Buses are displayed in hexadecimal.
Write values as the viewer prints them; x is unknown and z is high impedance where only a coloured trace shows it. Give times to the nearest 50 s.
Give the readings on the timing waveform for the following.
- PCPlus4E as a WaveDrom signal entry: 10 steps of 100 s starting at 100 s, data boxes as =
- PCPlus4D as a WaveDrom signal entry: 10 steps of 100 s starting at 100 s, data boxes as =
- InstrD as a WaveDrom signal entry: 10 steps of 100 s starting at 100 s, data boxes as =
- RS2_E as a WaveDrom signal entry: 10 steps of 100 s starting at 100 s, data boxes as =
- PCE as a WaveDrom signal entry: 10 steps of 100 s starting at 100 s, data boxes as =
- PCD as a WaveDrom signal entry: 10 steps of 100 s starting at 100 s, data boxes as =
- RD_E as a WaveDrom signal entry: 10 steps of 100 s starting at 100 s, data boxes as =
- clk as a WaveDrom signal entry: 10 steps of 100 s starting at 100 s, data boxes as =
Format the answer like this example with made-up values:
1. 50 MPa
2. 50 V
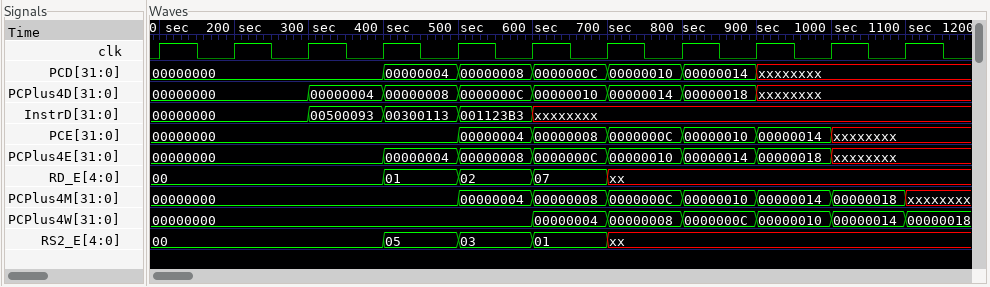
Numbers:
1. {name: 'PCPlus4E', wave: '=..======x', data: '00000000 00000004 00000008 0000000C 00000010 00000014 00000018'}
2. {name: 'PCPlus4D', wave: '=.======x.', data: '00000000 00000004 00000008 0000000C 00000010 00000014 00000018'}
3. {name: 'InstrD', wave: '=.===x....', data: '00000000 00500093 00300113 001123B3'}
4. {name: 'RS2_E', wave: '=..===x...', data: '00 05 03 01'}
5. {name: 'PCE', wave: '=...=====x', data: '00000000 00000004 00000008 0000000C 00000010 00000014'}
6. {name: 'PCD', wave: '=..=====x.', data: '00000000 00000004 00000008 0000000C 00000010 00000014'}
7. {name: 'RD_E', wave: '=..===x...', data: '00 01 02 07'}
8. {name: 'clk', wave: 'p.........'}
